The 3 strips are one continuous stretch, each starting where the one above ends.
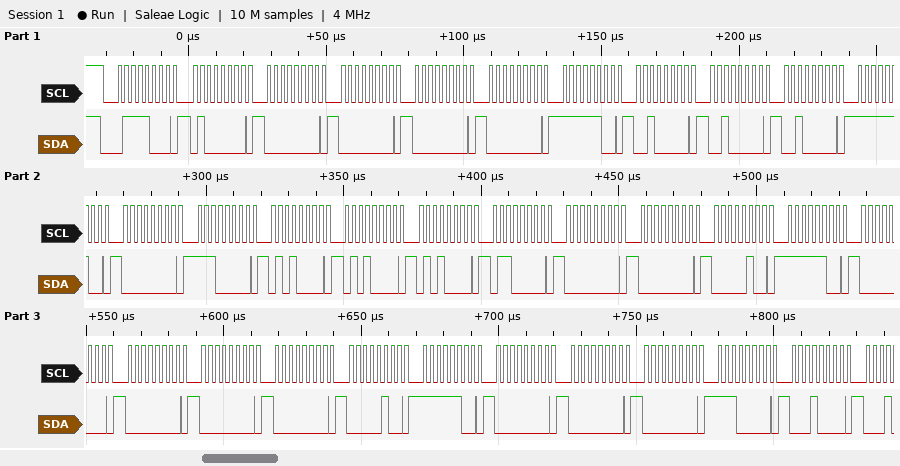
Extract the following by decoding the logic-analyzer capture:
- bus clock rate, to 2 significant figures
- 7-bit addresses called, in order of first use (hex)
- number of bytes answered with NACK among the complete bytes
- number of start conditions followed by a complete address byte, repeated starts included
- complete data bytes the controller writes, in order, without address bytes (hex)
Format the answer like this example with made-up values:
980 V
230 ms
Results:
400 kHz
0x3C
0
1
40 00 00 00 00 FC 20 20 20 FC 00 E0 50 50 50 60 00 00 04 FC 00 00 00 00 04 FC 00 00 00 E0 10
